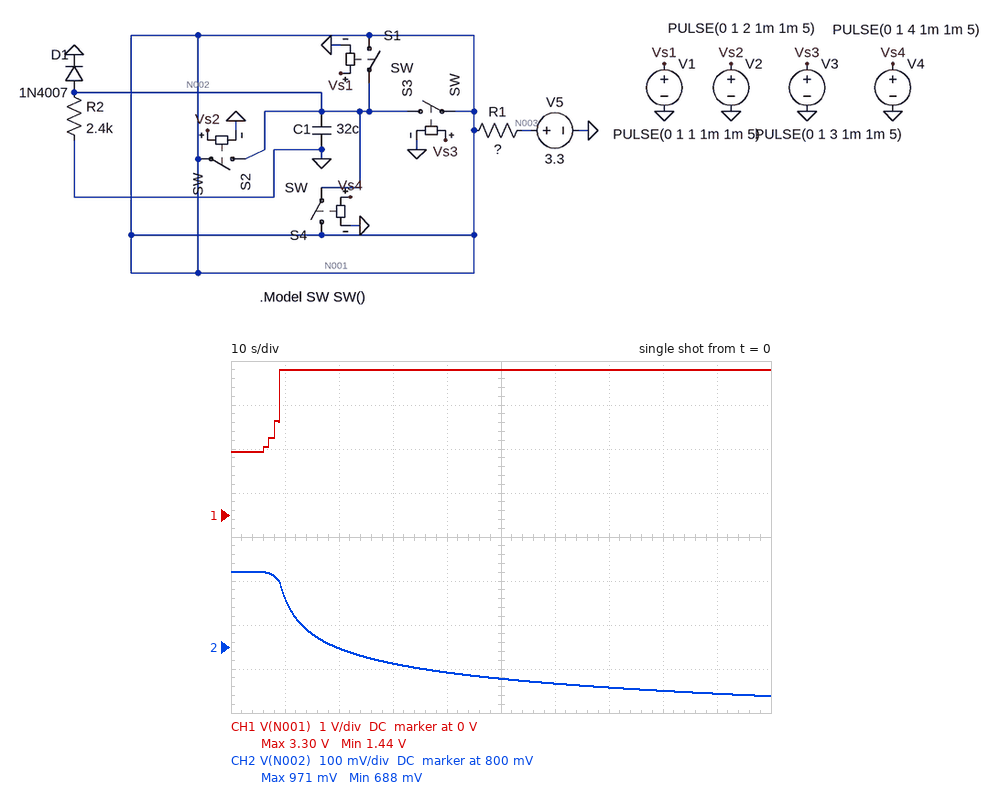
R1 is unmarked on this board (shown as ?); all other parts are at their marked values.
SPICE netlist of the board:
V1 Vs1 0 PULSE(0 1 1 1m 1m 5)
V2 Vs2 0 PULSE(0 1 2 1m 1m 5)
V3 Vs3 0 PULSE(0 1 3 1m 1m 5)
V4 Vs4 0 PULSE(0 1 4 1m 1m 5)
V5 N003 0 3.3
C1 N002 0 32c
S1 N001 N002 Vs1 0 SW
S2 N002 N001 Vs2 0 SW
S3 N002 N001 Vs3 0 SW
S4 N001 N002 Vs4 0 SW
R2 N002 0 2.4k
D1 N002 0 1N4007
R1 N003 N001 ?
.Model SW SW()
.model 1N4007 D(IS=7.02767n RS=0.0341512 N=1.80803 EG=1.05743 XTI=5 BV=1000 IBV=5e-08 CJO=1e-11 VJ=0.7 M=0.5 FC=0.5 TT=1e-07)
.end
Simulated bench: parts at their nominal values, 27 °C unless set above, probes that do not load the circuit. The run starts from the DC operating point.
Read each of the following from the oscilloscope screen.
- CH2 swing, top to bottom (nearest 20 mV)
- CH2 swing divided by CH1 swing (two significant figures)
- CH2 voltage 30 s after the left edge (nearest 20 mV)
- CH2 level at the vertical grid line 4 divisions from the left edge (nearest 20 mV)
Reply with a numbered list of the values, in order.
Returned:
1. 280 mV
2. 0.15
3. 760 mV
4. 740 mV
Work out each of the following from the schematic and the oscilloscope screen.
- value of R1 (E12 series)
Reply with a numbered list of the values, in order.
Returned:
1. 1 Ω
